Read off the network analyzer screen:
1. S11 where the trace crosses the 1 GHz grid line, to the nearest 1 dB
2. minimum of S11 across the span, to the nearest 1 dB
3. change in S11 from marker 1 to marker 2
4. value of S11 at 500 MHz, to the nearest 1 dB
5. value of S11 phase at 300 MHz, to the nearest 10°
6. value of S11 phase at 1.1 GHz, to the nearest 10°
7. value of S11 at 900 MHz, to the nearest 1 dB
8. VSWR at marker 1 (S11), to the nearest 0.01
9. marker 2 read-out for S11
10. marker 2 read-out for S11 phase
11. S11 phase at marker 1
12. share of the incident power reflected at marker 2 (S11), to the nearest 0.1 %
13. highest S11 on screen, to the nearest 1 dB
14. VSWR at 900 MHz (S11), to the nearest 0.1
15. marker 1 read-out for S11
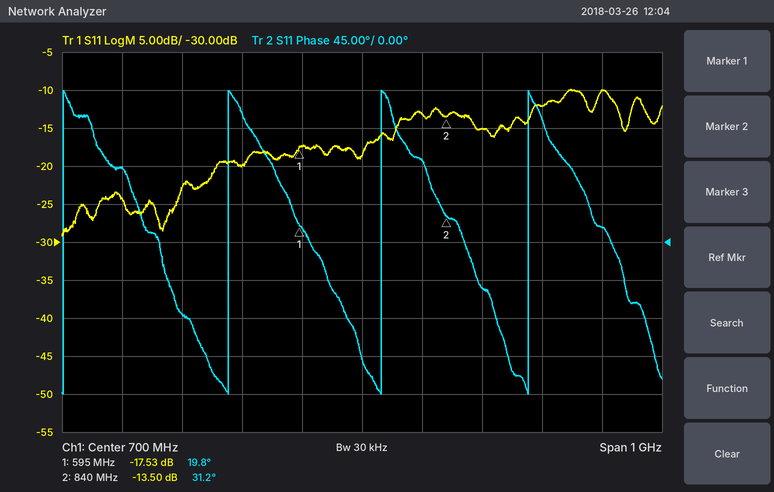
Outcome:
-12 dB
-29 dB
4.03 dB
-20 dB
90°
20°
-15 dB
1.31
-13.50 dB
31.2°
19.8°
4.5 %
-10 dB
1.4
-17.53 dB
